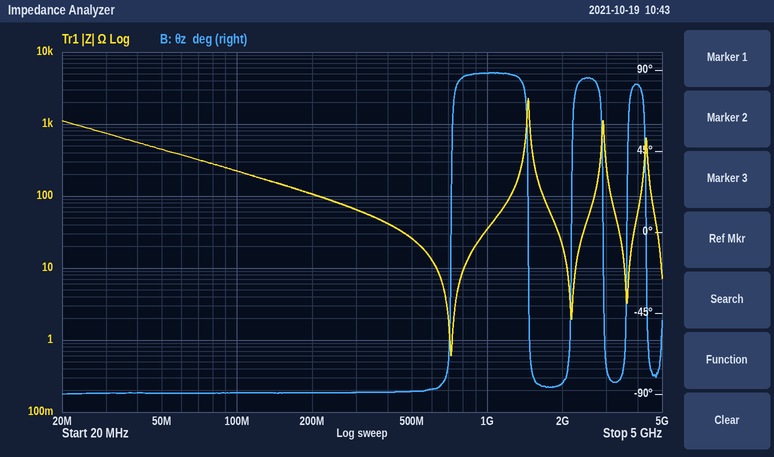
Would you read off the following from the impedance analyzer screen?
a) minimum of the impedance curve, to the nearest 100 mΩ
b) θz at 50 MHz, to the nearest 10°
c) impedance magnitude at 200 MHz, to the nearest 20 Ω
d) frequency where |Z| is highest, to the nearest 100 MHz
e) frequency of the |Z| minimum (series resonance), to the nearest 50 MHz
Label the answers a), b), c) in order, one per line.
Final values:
a) 600 mΩ
b) -90°
c) 100 Ω
d) 1.5 GHz
e) 700 MHz
